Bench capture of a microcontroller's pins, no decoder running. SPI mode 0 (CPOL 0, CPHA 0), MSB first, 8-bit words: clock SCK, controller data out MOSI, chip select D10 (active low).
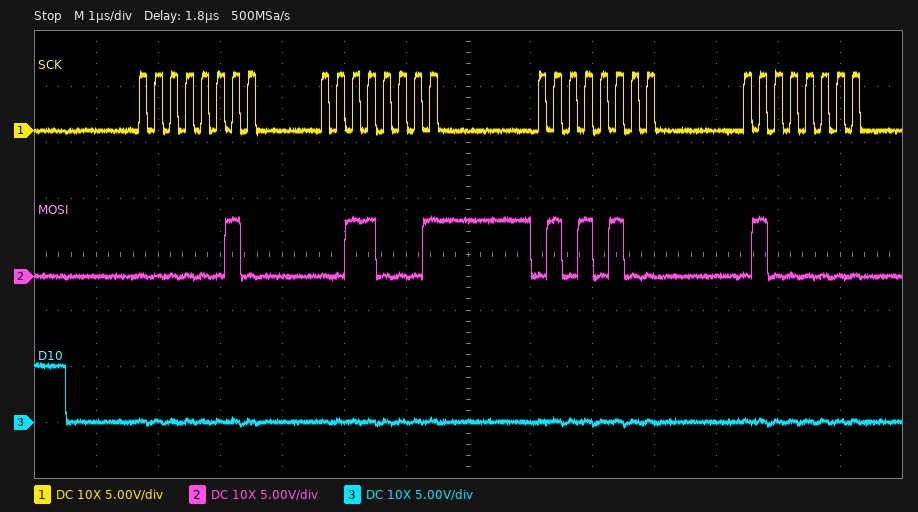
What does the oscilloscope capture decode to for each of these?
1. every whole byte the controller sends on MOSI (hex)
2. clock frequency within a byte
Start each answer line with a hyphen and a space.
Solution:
- 02 31 54 40
- 4 MHz
